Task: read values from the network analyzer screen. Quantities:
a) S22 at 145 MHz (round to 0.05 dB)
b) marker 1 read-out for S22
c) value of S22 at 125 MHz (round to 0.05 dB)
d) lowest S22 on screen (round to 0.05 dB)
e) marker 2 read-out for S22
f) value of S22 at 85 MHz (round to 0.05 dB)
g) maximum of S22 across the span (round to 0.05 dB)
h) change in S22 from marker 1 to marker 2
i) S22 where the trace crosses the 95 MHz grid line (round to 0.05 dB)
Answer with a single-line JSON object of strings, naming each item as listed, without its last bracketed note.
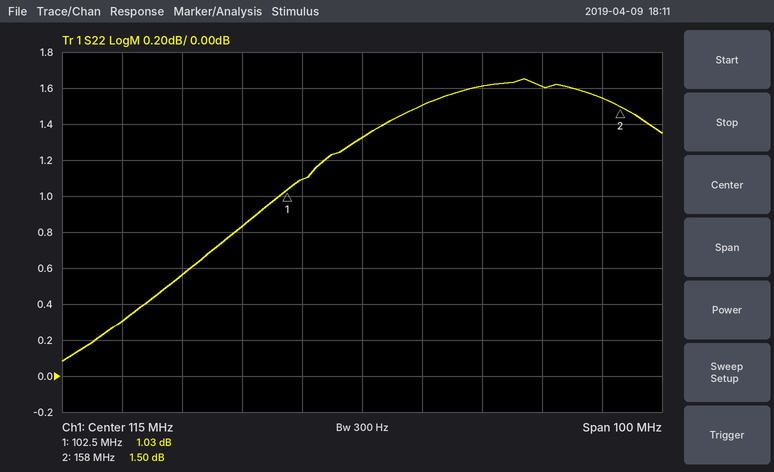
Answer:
{"S22 at 145 MHz": "1.60 dB", "marker 1 read-out for S22": "1.03 dB", "value of S22 at 125 MHz": "1.50 dB", "lowest S22 on screen": "0.10 dB", "marker 2 read-out for S22": "1.50 dB", "value of S22 at 85 MHz": "0.55 dB", "maximum of S22 across the span": "1.65 dB", "change in S22 from marker 1 to marker 2": "0.47 dB", "S22 where the trace crosses the 95 MHz grid line": "0.85 dB"}
